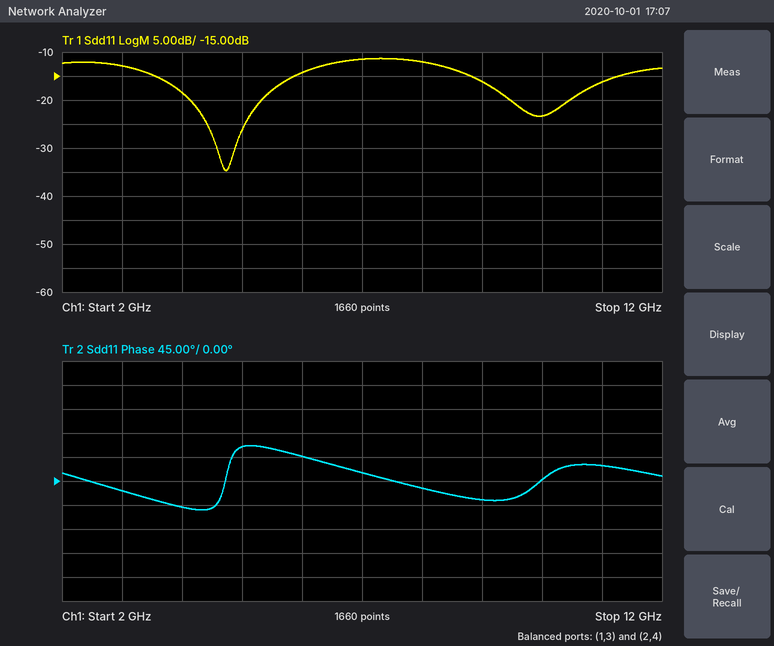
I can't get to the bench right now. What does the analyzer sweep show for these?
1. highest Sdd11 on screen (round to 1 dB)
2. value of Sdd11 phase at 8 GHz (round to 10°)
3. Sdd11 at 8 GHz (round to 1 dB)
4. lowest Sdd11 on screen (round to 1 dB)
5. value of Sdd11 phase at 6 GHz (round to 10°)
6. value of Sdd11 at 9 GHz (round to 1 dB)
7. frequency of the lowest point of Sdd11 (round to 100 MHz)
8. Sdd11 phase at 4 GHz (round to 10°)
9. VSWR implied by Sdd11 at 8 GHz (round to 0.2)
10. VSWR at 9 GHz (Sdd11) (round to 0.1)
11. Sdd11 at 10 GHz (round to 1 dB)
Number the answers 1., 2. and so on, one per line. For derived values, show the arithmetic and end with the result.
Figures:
1. -11 dB
2. -10°
3. -12 dB
4. -35 dB
5. 50°
6. -16 dB
7. 4.7 GHz
8. -50°
9. |Γ| = 10^(-12/20) = 0.2512; VSWR = (1 + 0.2512)/(1 − 0.2512) ≈ 1.67, so 1.6 to the nearest 0.2
10. |Γ| = 10^(-16/20) = 0.1585; VSWR = (1 + 0.1585)/(1 − 0.1585) ≈ 1.4
11. -23 dB
